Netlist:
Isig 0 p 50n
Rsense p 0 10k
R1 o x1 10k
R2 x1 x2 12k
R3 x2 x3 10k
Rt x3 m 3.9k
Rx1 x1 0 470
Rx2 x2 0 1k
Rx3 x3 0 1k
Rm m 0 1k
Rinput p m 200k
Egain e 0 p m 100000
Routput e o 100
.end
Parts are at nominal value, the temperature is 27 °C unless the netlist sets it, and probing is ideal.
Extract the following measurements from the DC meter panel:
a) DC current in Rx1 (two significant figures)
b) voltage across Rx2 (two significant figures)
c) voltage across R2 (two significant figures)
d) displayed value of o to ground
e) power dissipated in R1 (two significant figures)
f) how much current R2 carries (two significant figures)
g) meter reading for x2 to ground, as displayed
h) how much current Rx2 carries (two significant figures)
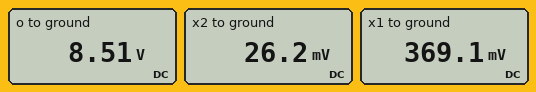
790 µA
26 mV
340 mV
8.51 V
6.6 mW
29 µA
26.2 mV
26 µA
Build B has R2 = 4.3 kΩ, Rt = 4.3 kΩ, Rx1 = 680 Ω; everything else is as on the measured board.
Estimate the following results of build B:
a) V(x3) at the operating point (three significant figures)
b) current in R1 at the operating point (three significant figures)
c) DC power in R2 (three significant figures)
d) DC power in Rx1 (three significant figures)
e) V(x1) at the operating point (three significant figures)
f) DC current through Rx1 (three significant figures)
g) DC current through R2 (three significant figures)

2.47 mV
301 µA
5.20 µW
48.3 µW
181 mV
267 µA
34.8 µA
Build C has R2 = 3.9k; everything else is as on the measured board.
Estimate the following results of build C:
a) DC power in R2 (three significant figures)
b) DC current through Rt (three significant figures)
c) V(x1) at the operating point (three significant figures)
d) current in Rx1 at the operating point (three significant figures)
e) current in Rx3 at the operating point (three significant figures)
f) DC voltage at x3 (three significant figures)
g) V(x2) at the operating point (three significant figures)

4.02 µW
460 nA
155 mV
329 µA
2.25 µA
2.25 mV
29.4 mV
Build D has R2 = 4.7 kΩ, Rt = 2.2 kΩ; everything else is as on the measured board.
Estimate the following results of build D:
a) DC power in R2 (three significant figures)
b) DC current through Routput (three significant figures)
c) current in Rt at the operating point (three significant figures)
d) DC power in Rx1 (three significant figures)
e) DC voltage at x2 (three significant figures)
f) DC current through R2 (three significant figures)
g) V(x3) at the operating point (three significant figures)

2.50 µW
299 µA
467 nA
35.7 µW
21.1 mV
23.1 µA
1.49 mV
